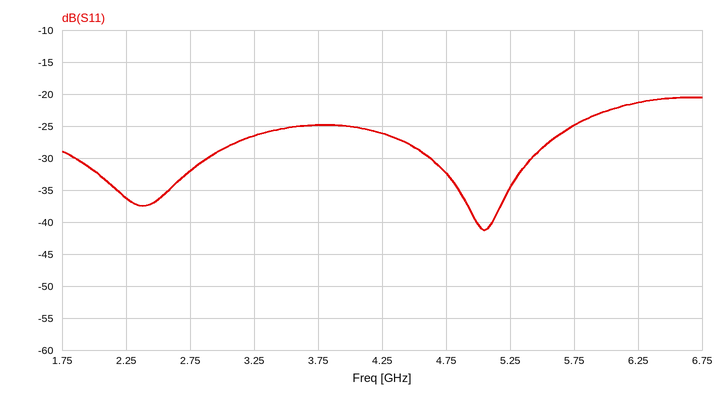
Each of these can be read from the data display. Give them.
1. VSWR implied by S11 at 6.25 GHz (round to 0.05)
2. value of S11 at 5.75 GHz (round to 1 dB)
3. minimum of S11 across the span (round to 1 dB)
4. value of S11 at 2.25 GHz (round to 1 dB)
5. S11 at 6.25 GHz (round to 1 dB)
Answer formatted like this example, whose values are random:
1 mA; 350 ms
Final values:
1.20; -25 dB; -41 dB; -36 dB; -21 dB
